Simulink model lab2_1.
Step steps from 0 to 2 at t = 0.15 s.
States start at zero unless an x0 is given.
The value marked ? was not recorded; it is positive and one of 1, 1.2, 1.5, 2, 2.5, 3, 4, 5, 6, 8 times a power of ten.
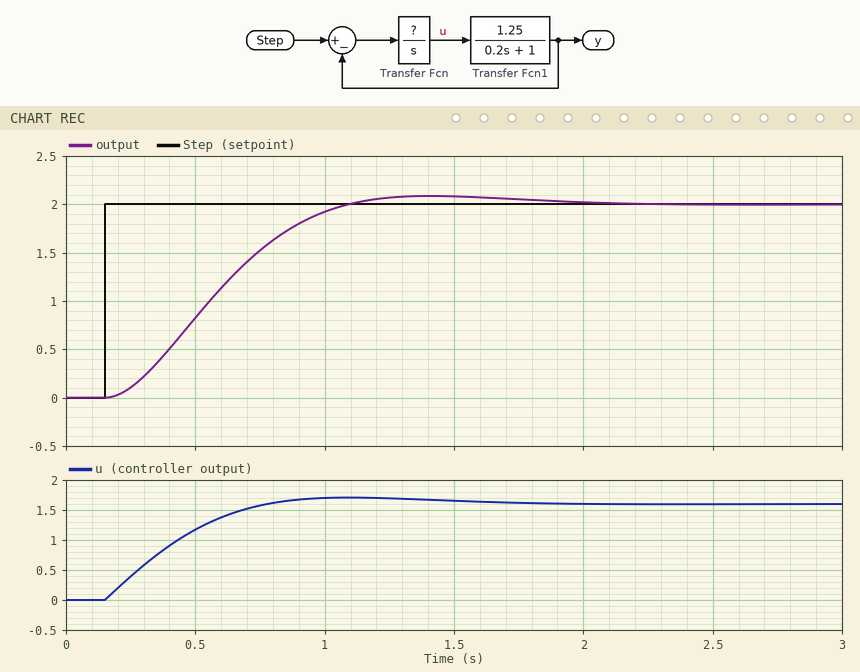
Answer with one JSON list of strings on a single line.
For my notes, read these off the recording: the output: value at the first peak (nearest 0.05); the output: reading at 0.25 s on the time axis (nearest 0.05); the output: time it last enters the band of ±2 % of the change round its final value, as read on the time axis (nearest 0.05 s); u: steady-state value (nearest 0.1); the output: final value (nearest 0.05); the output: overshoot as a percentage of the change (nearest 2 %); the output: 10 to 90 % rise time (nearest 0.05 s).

["2.10", "0.10", "1.85 s", "1.6", "2.00", "4 %", "0.60 s"]
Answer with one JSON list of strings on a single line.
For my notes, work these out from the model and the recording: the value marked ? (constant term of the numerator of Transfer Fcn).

["2"]
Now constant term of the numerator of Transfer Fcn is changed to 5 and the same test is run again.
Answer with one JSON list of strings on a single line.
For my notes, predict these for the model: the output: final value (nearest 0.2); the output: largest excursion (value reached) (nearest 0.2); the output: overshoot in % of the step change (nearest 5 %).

["2.0", "2.4", "20 %"]
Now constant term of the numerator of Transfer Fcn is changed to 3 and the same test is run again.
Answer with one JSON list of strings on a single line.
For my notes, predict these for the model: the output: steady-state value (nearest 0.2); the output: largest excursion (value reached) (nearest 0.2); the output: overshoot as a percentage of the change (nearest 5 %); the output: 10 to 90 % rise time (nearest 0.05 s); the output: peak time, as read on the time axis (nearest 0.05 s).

["2.0", "2.2", "10 %", "0.40 s", "1.05 s"]
